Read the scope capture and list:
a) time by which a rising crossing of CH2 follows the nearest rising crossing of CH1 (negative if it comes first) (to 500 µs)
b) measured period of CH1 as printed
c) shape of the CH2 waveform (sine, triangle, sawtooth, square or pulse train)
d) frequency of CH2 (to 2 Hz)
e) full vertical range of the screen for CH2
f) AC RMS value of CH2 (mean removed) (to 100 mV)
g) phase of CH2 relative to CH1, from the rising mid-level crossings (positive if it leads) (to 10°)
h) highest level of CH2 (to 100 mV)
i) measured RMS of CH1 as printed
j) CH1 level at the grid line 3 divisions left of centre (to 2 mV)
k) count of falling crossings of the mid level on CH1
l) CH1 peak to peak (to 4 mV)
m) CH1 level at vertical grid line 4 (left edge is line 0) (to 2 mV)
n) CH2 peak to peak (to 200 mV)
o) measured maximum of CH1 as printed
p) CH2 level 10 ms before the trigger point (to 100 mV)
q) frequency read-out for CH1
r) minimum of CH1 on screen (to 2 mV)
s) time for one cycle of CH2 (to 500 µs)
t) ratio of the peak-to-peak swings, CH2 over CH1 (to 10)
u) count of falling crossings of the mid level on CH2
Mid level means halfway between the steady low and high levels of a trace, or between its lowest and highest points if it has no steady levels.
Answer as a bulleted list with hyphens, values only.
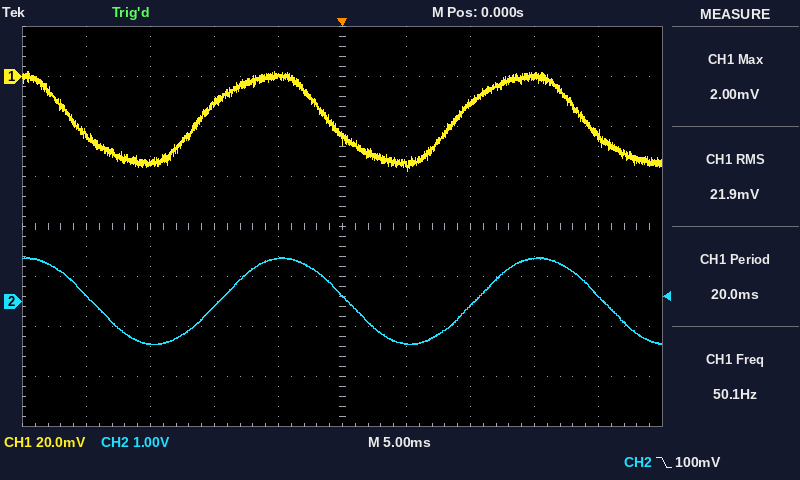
- +1.5 ms
- 20.0 ms
- sine
- 50 Hz
- 8 V
- 600 mV
- -30°
- 900 mV
- 21.9 mV
- -34 mV
- 3
- 40 mV
- 0 mV
- 1.8 V
- 2.00 mV
- -100 mV
- 50.1 Hz
- -38 mV
- 20.0 ms
- 40
- 3
